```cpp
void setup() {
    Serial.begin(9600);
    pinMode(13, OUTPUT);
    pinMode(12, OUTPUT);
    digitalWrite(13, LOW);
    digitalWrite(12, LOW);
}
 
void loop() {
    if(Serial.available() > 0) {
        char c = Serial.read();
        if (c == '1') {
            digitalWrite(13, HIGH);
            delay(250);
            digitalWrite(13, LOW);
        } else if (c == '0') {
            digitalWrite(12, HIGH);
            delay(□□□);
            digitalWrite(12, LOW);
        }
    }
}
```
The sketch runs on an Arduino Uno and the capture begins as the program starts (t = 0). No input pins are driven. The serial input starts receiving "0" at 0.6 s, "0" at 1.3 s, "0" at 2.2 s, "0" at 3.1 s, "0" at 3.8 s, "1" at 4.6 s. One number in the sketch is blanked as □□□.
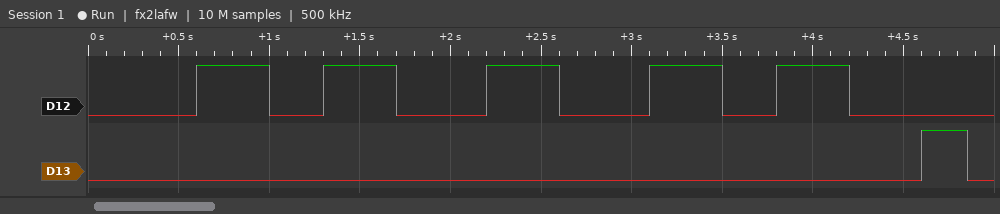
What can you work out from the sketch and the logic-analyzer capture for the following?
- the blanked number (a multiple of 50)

400
